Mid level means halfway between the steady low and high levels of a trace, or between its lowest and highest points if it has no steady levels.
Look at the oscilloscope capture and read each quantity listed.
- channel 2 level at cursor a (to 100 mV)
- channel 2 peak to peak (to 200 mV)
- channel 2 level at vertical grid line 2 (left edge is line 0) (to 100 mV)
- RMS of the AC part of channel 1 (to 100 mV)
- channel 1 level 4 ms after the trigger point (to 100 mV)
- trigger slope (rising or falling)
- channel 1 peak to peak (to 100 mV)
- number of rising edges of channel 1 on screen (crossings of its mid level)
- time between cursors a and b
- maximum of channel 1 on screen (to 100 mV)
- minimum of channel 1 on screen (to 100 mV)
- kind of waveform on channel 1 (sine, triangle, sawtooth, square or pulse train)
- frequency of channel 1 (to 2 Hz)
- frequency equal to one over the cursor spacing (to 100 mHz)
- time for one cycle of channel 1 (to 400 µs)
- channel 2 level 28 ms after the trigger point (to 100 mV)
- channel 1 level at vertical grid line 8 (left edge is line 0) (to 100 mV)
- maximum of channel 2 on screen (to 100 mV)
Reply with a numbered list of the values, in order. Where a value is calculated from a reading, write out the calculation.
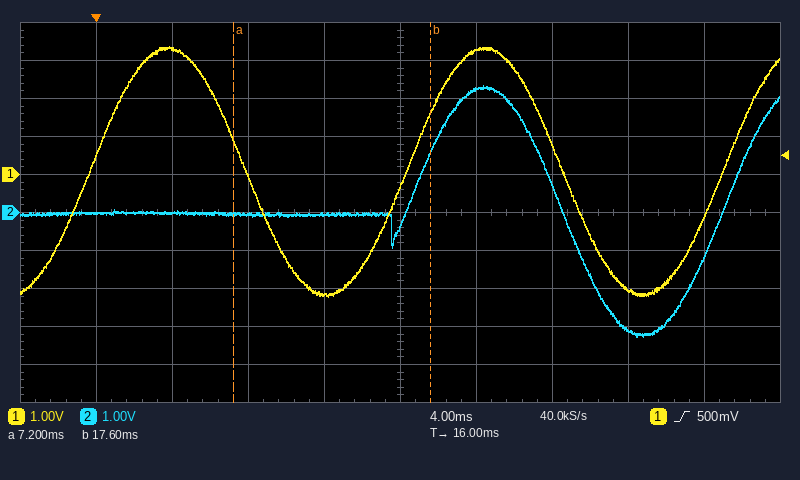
1. 0.0 V
2. 6.6 V
3. 0.0 V
4. 6.6 V / (2√2) ≈ 2.3 V
5. 3.3 V
6. rising
7. 3.4 V − (-3.2 V) = 6.6 V
8. 3
9. 17.6 ms − (7.2 ms) = 10.4 ms
10. 3.4 V
11. -3.2 V
12. sine
13. 1 / 16.8 ms ≈ 60 Hz
14. 1 / 10.4 ms ≈ 96.2 Hz
15. 16.8 ms
16. -3.1 V
17. -3.0 V
18. 3.3 V
